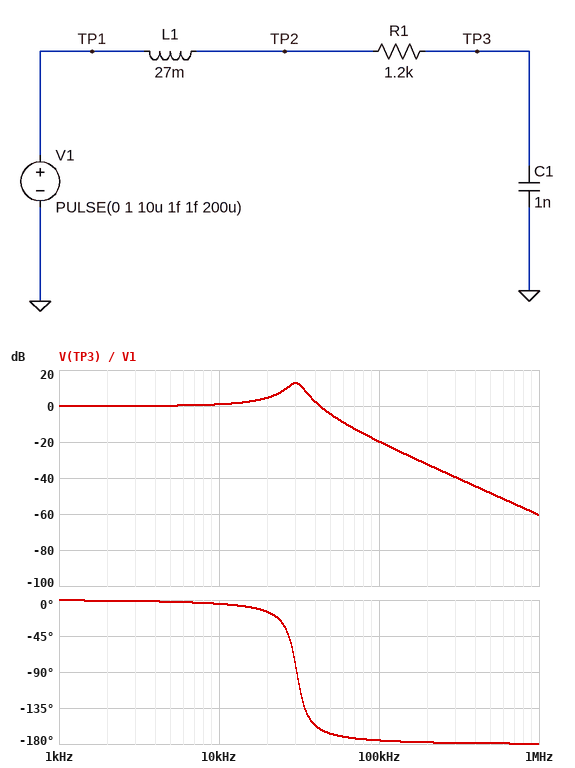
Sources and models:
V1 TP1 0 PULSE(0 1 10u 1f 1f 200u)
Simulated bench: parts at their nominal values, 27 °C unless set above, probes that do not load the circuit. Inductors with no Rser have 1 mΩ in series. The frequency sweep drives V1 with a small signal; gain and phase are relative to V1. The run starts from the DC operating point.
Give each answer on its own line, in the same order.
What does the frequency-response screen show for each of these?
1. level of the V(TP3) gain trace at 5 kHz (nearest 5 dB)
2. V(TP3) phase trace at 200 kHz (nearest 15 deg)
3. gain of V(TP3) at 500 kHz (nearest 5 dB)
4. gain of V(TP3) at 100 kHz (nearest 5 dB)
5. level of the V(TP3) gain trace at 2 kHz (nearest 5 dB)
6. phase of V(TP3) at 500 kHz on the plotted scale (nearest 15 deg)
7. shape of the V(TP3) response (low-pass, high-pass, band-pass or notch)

0 dB
-180 deg
-50 dB
-20 dB
0 dB
-180 deg
low-pass
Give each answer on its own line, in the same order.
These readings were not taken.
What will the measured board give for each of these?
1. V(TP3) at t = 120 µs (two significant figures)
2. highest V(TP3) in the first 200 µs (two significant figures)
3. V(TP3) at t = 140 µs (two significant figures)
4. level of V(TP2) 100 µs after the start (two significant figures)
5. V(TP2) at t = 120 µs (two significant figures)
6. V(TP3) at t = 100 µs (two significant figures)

1.0 V
1.7 V
950 mV
990 mV
1.1 V
1.0 V
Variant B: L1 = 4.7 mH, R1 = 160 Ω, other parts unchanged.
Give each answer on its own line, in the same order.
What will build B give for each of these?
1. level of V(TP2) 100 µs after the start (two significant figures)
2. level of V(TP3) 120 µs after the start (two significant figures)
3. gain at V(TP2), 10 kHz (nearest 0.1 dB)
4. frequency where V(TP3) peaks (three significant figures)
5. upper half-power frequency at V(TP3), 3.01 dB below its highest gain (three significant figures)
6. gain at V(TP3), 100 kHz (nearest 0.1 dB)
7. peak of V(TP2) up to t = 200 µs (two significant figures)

1.2 V
860 mV
0.2 dB
73.3 kHz
76.0 kHz
1.3 dB
1.9 V
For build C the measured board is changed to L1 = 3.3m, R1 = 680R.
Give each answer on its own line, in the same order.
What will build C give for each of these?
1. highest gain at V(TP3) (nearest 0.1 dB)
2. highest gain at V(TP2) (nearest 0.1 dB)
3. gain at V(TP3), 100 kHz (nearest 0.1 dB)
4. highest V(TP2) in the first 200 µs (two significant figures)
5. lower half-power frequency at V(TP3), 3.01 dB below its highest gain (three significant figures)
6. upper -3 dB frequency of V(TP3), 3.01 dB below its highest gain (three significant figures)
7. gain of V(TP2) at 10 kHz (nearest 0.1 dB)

8.7 dB
9.2 dB
5.6 dB
1.6 V
65.7 kHz
99.8 kHz
0.1 dB
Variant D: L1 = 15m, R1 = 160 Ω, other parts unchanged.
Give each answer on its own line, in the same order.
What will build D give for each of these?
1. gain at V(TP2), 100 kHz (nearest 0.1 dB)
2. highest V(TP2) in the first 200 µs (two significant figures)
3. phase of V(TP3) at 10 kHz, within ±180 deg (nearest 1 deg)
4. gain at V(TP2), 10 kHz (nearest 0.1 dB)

-13.8 dB
1.9 V
-1 deg
0.5 dB
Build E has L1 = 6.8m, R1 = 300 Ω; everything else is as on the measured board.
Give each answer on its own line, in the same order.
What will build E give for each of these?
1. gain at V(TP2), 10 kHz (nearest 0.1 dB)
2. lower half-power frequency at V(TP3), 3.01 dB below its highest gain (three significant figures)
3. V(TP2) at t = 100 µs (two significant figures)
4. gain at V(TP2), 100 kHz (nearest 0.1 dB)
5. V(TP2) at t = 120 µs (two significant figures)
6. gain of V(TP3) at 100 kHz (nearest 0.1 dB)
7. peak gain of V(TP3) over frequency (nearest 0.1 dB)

0.2 dB
57.2 kHz
1.1 V
-4.4 dB
1.0 V
-4.6 dB
18.8 dB
